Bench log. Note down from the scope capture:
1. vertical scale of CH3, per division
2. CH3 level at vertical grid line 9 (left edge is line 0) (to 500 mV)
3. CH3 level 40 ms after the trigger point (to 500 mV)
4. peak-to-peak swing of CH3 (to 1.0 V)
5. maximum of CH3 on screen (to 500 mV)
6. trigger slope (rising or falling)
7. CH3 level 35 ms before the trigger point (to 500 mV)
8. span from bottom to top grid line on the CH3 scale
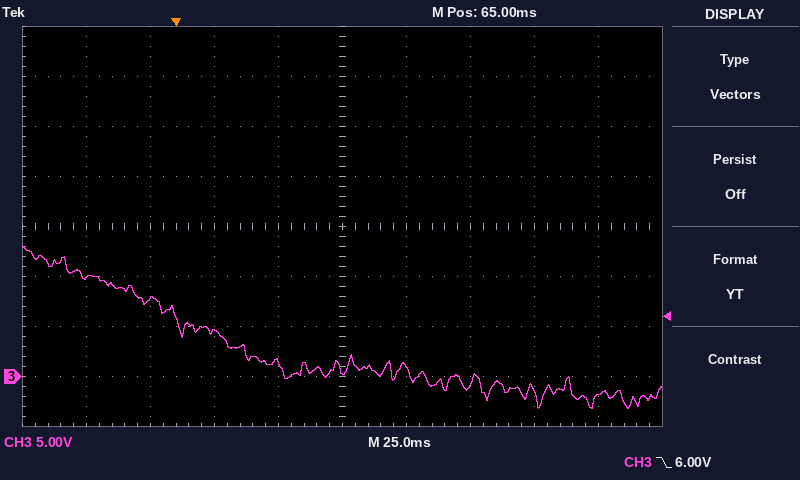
5 V
-2.0 V
1.5 V
16.0 V
13.0 V
falling
10.0 V
40 V
